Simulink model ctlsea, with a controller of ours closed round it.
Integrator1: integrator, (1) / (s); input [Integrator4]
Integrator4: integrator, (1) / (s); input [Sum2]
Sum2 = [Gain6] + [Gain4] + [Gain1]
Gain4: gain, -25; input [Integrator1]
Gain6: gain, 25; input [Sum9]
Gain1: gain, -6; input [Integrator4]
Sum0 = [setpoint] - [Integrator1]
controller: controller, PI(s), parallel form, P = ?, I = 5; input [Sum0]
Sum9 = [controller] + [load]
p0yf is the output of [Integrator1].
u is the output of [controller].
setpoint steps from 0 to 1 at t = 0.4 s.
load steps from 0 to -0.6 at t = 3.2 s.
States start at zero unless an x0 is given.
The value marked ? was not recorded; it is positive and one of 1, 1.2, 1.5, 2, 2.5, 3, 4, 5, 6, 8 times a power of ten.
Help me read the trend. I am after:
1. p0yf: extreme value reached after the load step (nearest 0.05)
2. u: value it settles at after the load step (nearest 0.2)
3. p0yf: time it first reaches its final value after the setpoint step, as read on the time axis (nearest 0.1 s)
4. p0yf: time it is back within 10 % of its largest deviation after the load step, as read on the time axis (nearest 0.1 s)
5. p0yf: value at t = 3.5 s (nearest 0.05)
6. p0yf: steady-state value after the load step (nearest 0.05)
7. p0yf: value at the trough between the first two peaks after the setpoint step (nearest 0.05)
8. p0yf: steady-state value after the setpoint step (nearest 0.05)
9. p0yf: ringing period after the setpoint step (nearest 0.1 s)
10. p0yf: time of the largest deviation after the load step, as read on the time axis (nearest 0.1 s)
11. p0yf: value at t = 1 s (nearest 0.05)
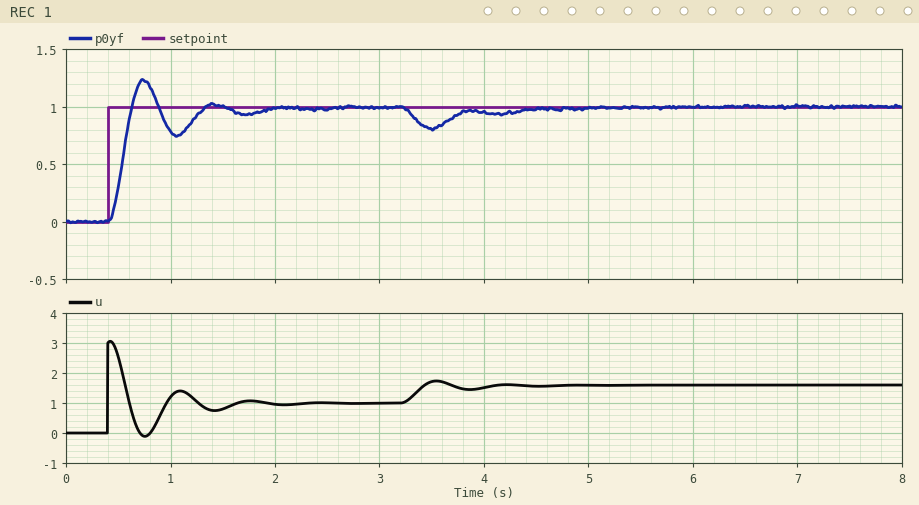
0.80
1.6
0.6 s
5.0 s
0.80
1.00
0.75
1.00
0.7 s
3.5 s
0.80
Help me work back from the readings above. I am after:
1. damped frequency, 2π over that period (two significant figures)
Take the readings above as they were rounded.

9.0 rad/s
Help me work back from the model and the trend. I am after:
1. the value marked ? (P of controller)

3
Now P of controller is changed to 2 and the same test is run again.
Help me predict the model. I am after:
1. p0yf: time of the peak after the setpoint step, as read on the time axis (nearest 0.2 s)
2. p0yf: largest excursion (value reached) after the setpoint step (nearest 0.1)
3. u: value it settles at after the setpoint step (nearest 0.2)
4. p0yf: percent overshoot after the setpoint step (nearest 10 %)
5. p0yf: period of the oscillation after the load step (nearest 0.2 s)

0.8 s
1.2
1.0
20 %
0.8 s
